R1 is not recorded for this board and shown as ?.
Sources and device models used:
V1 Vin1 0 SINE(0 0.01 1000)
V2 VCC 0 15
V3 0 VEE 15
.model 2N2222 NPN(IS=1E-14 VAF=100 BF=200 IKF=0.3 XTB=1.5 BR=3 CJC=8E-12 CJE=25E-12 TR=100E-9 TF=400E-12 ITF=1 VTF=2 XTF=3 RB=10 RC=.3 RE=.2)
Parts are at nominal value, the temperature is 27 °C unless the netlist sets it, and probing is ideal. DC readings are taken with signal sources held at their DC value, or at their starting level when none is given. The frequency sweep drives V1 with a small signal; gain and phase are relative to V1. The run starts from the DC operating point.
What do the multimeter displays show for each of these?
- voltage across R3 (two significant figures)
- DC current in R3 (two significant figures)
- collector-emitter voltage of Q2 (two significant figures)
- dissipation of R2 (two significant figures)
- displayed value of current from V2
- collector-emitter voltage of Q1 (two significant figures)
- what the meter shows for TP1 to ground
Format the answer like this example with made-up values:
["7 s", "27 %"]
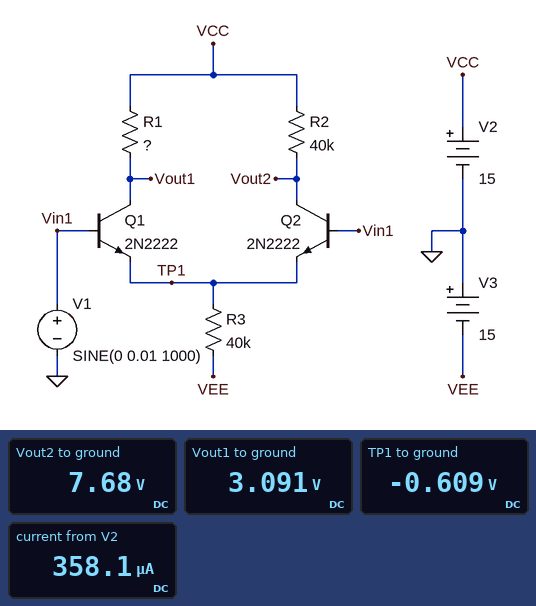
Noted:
["14 V", "360 µA", "8.3 V", "1.3 mW", "358.1 µA", "3.7 V", "-0.609 V"]
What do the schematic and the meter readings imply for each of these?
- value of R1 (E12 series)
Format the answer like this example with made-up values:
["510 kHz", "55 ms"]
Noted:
["68 kΩ"]
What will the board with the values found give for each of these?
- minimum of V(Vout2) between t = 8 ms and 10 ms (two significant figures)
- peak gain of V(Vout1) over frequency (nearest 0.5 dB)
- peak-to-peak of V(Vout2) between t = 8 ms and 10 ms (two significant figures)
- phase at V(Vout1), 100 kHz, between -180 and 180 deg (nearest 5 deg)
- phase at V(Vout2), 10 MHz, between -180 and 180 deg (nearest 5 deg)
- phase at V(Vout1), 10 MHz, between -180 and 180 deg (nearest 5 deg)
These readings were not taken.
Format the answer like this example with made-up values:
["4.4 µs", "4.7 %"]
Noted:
["7.7 V", "0 dB", "10 mV", "155 deg", "10 deg", "5 deg"]
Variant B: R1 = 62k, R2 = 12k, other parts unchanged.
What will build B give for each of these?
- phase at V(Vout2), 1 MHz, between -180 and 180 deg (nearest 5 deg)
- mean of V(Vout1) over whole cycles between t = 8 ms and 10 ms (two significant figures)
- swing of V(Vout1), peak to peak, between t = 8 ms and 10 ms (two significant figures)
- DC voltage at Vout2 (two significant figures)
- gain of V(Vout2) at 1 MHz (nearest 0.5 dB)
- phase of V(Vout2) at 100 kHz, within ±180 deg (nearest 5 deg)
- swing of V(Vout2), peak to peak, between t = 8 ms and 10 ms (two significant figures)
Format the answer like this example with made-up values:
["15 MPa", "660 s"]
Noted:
["110 deg", "4.3 V", "14 mV", "13 V", "-11.0 dB", "170 deg", "3.2 mV"]
